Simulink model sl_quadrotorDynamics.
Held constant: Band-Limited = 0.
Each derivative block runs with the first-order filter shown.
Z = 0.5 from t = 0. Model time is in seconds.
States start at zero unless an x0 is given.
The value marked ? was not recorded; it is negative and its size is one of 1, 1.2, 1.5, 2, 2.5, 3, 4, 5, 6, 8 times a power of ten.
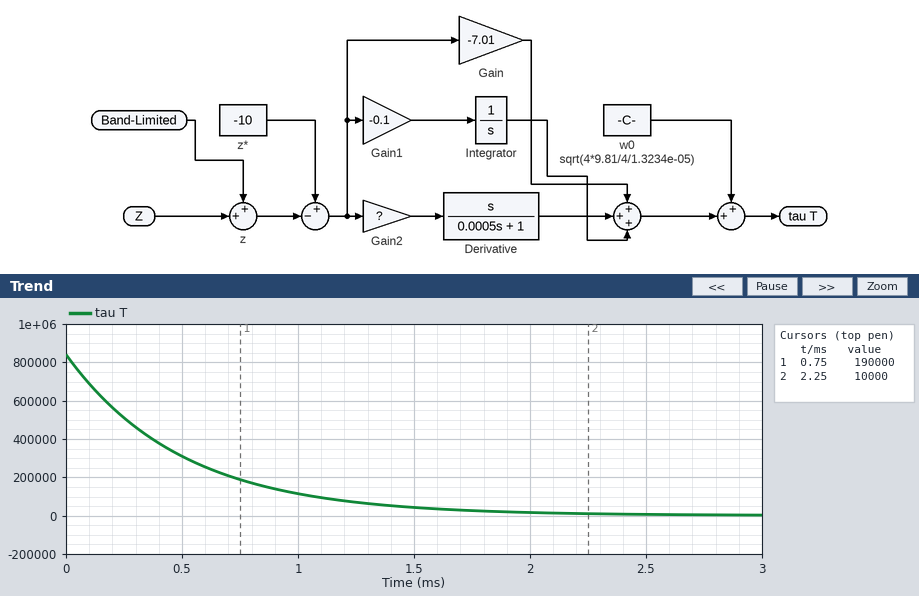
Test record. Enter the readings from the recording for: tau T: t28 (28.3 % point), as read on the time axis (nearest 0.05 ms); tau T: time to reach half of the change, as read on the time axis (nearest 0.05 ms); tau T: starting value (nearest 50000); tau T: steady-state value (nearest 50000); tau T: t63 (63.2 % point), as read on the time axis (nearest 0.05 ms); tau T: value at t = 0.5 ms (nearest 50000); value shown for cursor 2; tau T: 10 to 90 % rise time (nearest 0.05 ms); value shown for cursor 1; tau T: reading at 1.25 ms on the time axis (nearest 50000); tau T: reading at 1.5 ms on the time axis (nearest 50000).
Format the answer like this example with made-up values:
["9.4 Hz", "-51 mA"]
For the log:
["0.15 ms", "0.35 ms", "850000", "0", "0.50 ms", "300000", "10000", "1.10 ms", "190000", "50000", "50000"]
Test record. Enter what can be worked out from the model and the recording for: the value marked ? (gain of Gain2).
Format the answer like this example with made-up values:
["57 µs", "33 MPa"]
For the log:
["-40"]
